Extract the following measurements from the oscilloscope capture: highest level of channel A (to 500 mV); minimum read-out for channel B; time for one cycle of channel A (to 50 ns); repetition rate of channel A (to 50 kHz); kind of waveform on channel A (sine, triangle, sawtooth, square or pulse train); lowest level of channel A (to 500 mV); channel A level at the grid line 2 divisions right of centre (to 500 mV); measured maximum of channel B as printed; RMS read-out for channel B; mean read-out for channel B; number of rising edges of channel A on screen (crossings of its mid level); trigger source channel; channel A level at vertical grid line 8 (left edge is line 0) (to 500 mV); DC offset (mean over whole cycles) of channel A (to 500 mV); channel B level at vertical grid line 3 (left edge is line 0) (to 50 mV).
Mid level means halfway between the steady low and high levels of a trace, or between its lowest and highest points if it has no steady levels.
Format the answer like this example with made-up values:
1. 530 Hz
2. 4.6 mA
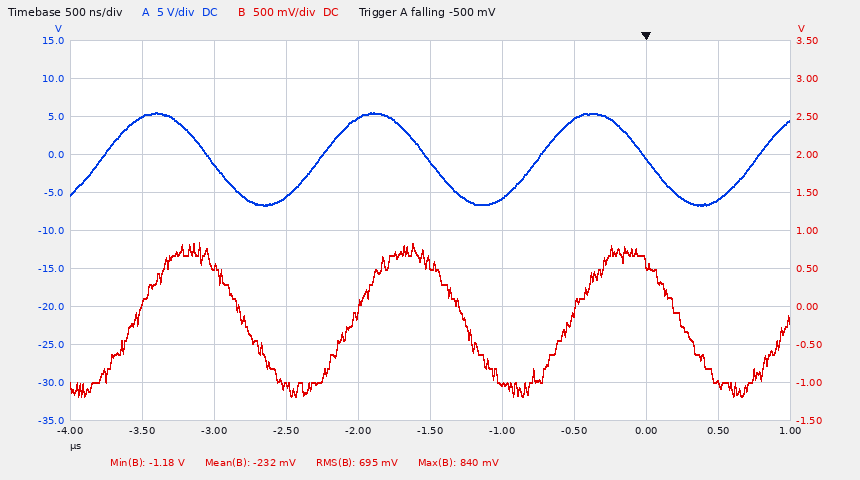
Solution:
1. 5.5 V
2. -1.18 V
3. 1.50 µs
4. 650 kHz
5. sine
6. -6.5 V
7. 4.5 V
8. 840 mV
9. 695 mV
10. -232 mV
11. 4
12. channel A
13. -500 mV
14. -500 mV
15. -1.05 V
